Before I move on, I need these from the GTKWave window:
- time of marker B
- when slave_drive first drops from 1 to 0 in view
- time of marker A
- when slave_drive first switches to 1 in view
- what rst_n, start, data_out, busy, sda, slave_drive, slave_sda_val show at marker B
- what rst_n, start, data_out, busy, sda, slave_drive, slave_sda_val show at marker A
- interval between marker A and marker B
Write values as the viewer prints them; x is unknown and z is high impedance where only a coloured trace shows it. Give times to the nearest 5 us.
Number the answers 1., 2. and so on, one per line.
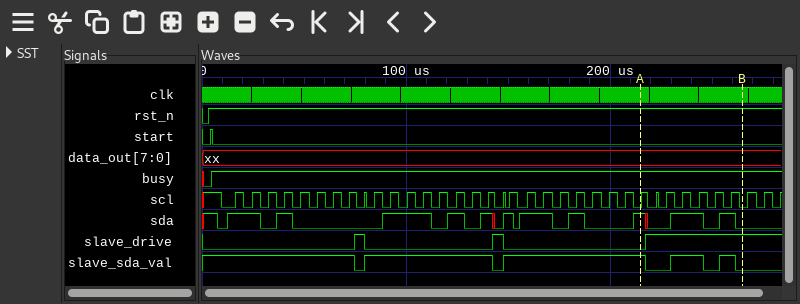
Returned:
1. 265 us
2. 80 us
3. 215 us
4. 75 us
5. rst_n=1, start=0, data_out=xx, busy=1, sda=0, slave_drive=1, slave_sda_val=0
6. rst_n=1, start=0, data_out=xx, busy=1, sda=1, slave_drive=0, slave_sda_val=1
7. 50 us
